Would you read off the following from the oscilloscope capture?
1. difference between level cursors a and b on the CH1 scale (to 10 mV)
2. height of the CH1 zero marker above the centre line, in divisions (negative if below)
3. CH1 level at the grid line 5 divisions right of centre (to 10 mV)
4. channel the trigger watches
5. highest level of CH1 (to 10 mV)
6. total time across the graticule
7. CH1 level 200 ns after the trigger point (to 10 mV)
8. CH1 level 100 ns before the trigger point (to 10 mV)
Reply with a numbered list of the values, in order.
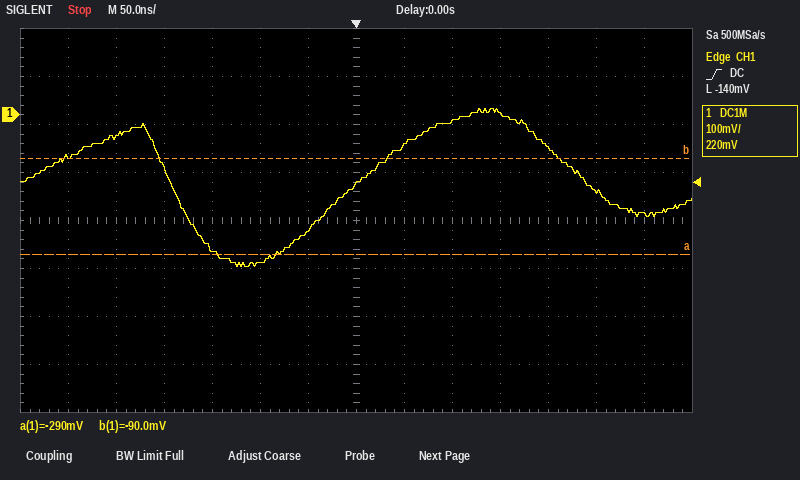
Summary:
1. 200 mV
2. +2.2 div
3. -160 mV
4. CH1
5. 10 mV
6. 700 ns
7. -70 mV
8. -310 mV
